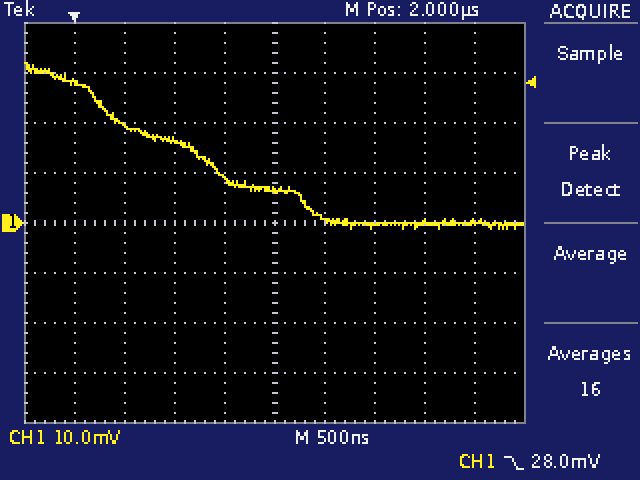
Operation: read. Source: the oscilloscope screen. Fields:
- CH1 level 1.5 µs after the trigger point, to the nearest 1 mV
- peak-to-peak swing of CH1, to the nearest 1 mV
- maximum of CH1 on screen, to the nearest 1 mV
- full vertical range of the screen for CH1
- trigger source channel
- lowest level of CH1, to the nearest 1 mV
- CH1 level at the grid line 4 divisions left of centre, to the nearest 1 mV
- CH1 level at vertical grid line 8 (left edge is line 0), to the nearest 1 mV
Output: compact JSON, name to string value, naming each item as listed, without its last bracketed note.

{"CH1 level 1.5 µs after the trigger point, to the nearest 1 mV": "9 mV", "peak-to-peak swing of CH1, to the nearest 1 mV": "33 mV", "maximum of CH1 on screen, to the nearest 1 mV": "32 mV", "full vertical range of the screen for CH1": "80 mV", "trigger source channel": "CH1", "lowest level of CH1, to the nearest 1 mV": "-1 mV", "CH1 level at the grid line 4 divisions left of centre, to the nearest 1 mV": "28 mV", "CH1 level at vertical grid line 8 (left edge is line 0), to the nearest 1 mV": "0 mV"}
